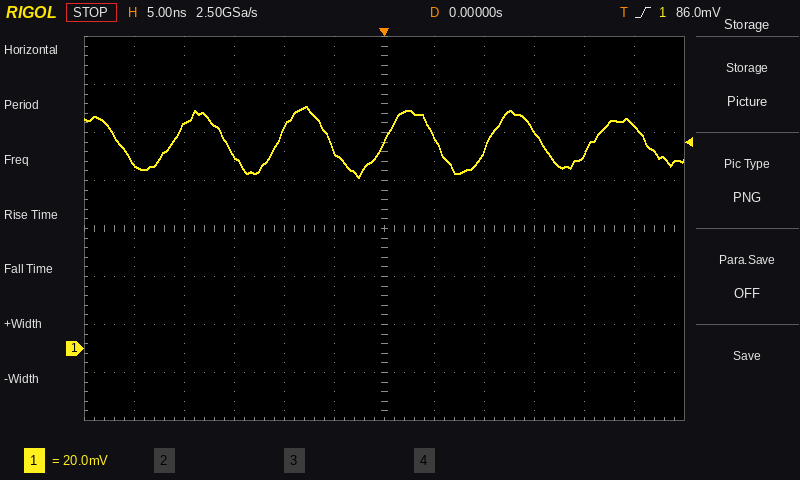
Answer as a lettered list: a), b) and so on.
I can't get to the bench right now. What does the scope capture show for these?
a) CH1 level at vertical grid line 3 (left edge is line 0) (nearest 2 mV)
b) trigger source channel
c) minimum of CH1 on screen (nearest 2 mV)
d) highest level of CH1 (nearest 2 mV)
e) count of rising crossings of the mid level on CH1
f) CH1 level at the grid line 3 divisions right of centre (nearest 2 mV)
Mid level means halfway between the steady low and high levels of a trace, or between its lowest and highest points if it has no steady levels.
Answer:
a) 80 mV
b) CH1
c) 72 mV
d) 100 mV
e) 5
f) 90 mV
